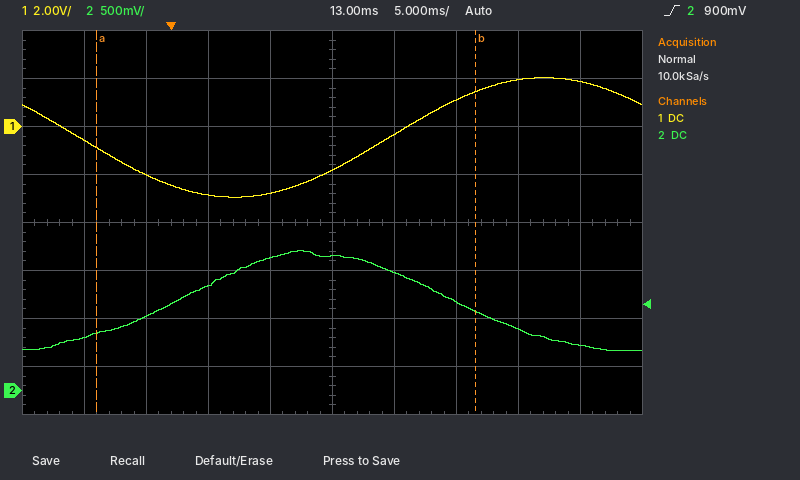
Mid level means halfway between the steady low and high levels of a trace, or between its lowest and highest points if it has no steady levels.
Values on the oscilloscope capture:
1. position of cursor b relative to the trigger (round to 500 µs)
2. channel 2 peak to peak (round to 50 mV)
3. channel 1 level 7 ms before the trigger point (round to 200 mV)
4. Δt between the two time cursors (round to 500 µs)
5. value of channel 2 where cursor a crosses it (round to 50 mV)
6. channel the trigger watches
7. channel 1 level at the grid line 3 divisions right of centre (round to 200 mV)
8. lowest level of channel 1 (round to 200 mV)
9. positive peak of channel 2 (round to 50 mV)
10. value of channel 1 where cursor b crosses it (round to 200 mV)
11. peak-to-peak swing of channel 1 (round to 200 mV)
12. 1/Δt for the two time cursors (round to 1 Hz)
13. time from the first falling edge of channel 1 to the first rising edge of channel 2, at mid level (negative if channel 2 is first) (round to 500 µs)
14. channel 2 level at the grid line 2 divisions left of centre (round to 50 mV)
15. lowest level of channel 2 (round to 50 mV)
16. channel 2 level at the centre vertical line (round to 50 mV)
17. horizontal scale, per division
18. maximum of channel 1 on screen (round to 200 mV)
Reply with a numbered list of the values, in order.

1. +24.5 ms
2. 1.05 V
3. -600 mV
4. 30.5 ms
5. 600 mV
6. channel 2
7. 2.0 V
8. -3.0 V
9. 1.45 V
10. 1.4 V
11. 5.0 V
12. 33 Hz
13. +8.0 ms
14. 1.10 V
15. 400 mV
16. 1.40 V
17. 5 ms
18. 2.0 V
